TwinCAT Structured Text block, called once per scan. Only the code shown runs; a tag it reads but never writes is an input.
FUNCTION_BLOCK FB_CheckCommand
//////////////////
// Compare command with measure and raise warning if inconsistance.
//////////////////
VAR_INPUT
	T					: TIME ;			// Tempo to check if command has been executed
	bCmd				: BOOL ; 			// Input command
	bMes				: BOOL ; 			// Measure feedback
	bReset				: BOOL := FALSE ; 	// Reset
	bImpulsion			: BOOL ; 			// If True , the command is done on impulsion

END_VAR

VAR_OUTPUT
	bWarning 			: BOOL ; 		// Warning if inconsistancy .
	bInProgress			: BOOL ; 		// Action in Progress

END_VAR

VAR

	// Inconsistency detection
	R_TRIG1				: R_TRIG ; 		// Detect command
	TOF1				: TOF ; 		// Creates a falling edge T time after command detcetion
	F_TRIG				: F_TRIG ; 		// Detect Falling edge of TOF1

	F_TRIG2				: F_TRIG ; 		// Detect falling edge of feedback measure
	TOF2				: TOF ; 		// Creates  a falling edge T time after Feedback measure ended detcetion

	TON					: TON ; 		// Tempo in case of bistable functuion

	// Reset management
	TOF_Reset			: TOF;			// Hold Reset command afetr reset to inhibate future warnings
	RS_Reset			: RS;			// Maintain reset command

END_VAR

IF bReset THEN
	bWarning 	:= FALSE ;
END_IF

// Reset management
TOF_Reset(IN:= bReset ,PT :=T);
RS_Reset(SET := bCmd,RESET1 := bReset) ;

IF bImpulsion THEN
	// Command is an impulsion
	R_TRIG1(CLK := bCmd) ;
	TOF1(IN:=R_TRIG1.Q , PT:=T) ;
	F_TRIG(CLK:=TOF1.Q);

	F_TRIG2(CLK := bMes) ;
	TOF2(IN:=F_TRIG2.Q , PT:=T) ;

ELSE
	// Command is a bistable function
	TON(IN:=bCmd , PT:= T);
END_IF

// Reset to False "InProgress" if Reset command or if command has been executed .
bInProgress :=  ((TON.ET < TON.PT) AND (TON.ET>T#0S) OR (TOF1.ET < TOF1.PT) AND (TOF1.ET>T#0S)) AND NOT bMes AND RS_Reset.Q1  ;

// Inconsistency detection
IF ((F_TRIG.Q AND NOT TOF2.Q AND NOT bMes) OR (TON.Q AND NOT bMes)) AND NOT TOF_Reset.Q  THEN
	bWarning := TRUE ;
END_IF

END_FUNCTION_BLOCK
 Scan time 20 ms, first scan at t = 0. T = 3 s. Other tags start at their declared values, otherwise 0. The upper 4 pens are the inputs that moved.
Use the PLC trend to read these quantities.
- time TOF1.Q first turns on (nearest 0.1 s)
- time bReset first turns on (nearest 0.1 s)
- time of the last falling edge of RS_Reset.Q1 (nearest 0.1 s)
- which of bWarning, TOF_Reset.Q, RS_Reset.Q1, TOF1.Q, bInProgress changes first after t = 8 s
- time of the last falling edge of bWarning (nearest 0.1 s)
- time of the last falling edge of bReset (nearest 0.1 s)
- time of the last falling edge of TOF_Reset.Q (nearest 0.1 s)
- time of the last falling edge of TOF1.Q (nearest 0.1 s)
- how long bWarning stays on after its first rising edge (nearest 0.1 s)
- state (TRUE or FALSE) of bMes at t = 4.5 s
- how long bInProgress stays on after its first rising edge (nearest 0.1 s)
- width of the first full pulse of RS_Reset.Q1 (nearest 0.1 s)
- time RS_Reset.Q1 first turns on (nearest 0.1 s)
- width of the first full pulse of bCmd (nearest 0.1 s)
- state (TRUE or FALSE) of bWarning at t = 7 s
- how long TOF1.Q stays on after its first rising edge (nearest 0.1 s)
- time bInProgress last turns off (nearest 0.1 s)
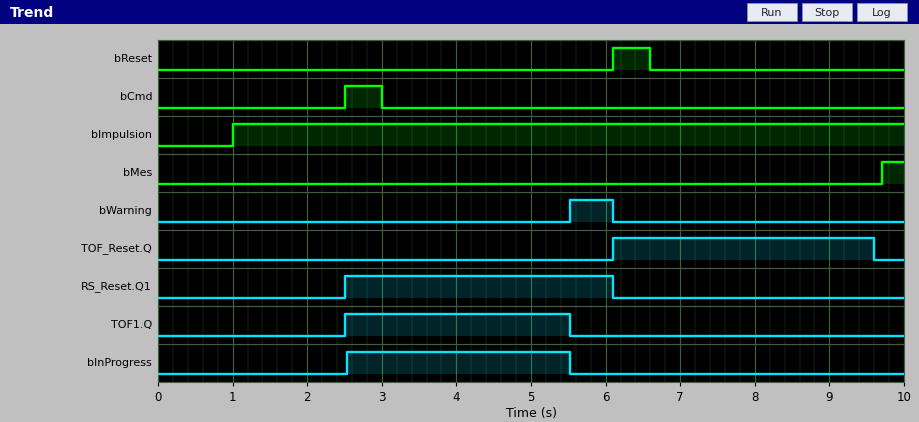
2.5 s
6.1 s
6.1 s
TOF_Reset.Q
6.1 s
6.6 s
9.6 s
5.5 s
0.6 s
FALSE
3.0 s
3.6 s
2.5 s
0.5 s
FALSE
3.0 s
5.5 s
